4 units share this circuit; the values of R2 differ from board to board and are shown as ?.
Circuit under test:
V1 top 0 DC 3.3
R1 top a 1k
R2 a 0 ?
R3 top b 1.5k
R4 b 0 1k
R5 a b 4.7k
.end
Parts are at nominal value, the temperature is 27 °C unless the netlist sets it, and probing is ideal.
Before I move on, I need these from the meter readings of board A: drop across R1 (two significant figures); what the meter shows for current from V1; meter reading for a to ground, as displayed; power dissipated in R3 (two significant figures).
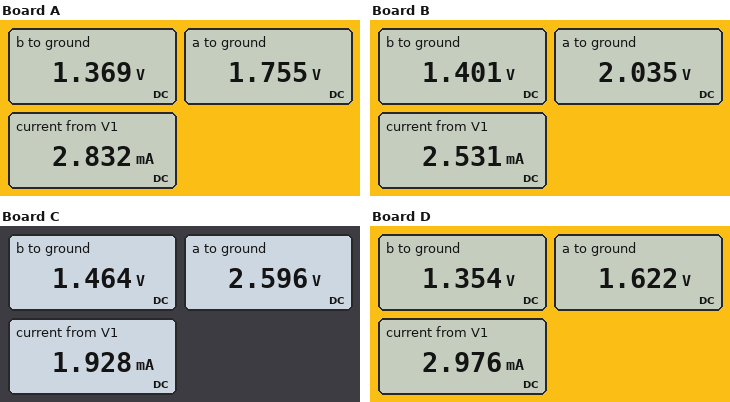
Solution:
1.5 V
2.832 mA
1.755 V
2.5 mW
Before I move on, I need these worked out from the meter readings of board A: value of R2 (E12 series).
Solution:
1.2 kΩ
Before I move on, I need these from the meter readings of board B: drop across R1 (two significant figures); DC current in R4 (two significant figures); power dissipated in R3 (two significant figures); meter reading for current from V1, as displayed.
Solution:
1.3 V
1.4 mA
2.4 mW
2.531 mA
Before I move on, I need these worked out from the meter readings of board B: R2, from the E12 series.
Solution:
1.8 kΩ
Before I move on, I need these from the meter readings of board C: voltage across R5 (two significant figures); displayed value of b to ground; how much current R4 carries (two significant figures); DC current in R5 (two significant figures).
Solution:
1.1 V
1.464 V
1.5 mA
240 µA
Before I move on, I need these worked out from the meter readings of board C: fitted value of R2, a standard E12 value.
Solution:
5.6 kΩ
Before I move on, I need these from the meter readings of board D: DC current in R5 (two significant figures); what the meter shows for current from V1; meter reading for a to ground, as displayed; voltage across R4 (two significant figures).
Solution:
57 µA
2.976 mA
1.622 V
1.4 V
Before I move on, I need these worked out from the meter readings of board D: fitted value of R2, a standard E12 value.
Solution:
1 kΩ
